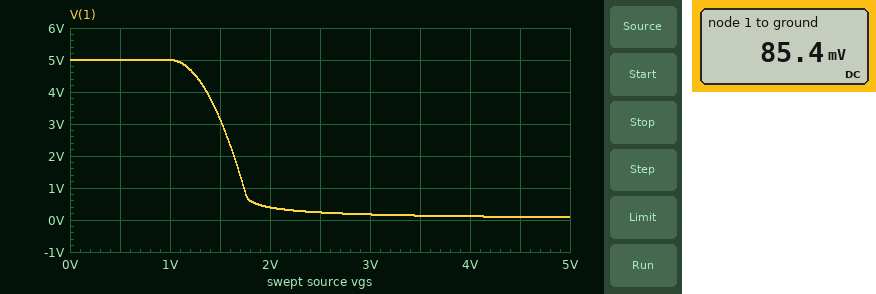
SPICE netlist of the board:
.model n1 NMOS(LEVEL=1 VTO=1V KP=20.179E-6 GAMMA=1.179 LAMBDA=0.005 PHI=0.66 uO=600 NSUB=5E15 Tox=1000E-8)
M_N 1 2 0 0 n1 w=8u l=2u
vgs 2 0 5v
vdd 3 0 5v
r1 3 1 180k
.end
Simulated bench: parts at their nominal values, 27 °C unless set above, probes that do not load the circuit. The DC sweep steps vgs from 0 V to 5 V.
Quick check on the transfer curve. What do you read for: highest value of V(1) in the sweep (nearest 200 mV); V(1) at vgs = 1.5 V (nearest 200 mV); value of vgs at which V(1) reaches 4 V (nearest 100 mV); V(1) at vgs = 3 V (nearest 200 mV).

5.0 V
3.2 V
1.4 V
200 mV
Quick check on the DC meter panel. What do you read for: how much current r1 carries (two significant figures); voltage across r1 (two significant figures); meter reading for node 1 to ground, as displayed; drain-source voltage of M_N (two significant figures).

27 µA
4.9 V
85.4 mV
85 mV
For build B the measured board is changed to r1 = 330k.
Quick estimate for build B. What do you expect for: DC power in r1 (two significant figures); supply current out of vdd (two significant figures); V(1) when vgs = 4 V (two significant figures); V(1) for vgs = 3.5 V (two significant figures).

74 µW
15 µA
62 mV
75 mV
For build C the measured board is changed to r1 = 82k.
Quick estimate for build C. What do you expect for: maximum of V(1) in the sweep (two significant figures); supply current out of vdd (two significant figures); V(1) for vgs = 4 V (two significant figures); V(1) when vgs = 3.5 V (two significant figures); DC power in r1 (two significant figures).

5.0 V
59 µA
250 mV
300 mV
280 µW
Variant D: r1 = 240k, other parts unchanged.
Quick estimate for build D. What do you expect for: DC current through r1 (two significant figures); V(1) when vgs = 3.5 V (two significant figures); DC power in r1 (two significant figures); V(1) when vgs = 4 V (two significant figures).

21 µA
100 mV
100 µW
86 mV
